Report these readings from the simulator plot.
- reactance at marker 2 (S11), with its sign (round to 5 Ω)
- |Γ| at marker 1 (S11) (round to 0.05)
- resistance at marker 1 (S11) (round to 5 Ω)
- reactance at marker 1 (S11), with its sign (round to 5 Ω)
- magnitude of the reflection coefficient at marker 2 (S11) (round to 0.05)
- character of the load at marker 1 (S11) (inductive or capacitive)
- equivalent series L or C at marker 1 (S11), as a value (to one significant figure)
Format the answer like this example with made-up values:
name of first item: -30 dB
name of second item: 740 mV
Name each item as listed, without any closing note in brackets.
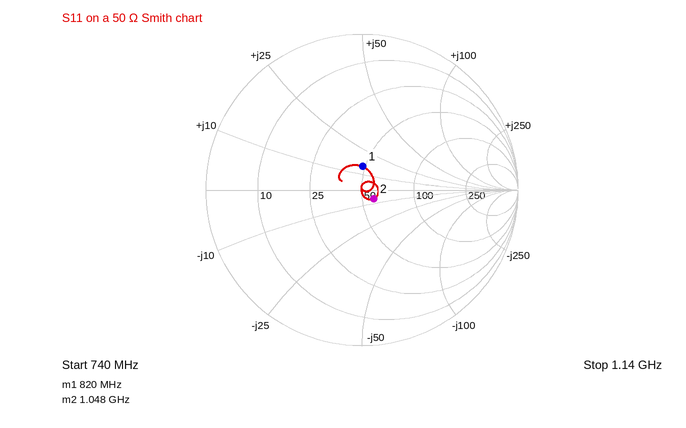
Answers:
reactance at marker 2 (S11), with its sign: -5 Ω
|Γ| at marker 1 (S11): 0.15
resistance at marker 1 (S11): 50 Ω
reactance at marker 1 (S11), with its sign: +15 Ω
magnitude of the reflection coefficient at marker 2 (S11): 0.10
character of the load at marker 1 (S11): inductive
equivalent series L or C at marker 1 (S11), as a value: 3 nH
